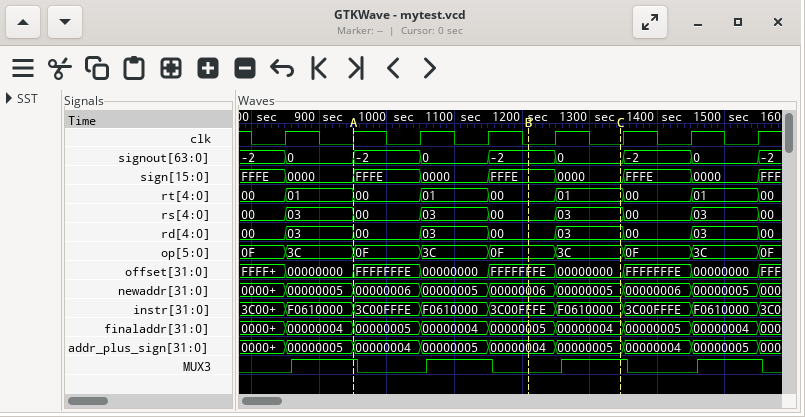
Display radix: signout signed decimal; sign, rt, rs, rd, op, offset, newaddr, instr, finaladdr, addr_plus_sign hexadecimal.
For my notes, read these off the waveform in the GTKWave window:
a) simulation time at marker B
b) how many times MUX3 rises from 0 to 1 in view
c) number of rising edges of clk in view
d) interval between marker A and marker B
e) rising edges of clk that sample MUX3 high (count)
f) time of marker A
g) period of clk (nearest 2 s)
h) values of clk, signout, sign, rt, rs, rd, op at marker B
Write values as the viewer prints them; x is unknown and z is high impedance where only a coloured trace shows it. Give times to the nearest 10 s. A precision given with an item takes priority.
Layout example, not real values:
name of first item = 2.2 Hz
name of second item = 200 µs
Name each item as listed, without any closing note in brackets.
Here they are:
simulation time at marker B = 1210 s
how many times MUX3 rises from 0 to 1 in view = 4
number of rising edges of clk in view = 8
interval between marker A and marker B = 260 s
rising edges of clk that sample MUX3 high = 4
time of marker A = 950 s
period of clk = 100 s
values of clk, signout, sign, rt, rs, rd, op at marker B = clk=0, signout=-2, sign=FFFE, rt=00, rs=00, rd=00, op=0F
